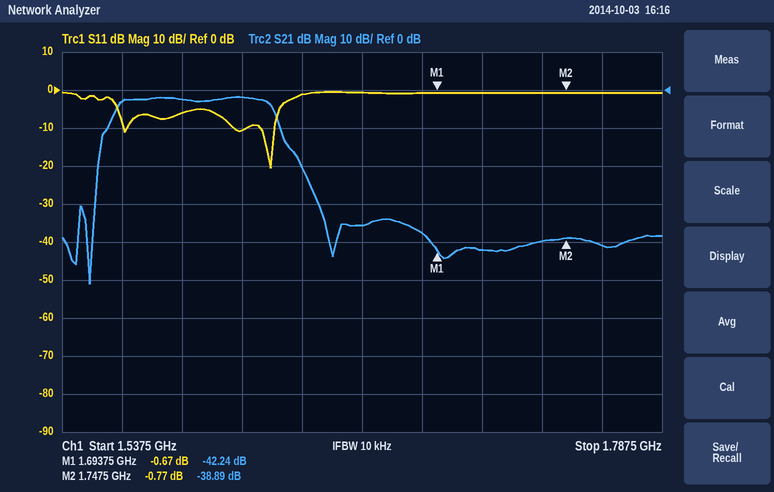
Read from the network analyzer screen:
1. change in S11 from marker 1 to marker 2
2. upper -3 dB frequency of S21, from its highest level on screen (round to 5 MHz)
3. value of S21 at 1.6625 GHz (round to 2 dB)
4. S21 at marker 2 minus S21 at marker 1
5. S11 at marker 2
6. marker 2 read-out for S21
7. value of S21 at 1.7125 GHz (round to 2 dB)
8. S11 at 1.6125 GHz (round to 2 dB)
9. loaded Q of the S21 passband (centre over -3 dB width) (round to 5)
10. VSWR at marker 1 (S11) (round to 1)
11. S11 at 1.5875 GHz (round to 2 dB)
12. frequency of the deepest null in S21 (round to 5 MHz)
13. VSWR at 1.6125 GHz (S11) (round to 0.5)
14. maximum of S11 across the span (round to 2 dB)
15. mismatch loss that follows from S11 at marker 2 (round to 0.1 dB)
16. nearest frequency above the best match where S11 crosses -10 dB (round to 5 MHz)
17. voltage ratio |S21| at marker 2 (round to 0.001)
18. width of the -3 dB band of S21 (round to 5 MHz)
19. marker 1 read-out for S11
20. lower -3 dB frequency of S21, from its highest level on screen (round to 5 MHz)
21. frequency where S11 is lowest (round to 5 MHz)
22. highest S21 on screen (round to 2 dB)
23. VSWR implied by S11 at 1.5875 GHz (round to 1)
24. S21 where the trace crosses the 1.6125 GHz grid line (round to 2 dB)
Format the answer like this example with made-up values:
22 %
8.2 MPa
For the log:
-0.10 dB
1.625 GHz
-36 dB
3.35 dB
-0.77 dB
-38.89 dB
-42 dB
-10 dB
25
26
-6 dB
1.550 GHz
2.0
0 dB
7.9 dB
1.625 GHz
0.011
65 MHz
-0.67 dB
1.560 GHz
1.625 GHz
-2 dB
3
-2 dB
